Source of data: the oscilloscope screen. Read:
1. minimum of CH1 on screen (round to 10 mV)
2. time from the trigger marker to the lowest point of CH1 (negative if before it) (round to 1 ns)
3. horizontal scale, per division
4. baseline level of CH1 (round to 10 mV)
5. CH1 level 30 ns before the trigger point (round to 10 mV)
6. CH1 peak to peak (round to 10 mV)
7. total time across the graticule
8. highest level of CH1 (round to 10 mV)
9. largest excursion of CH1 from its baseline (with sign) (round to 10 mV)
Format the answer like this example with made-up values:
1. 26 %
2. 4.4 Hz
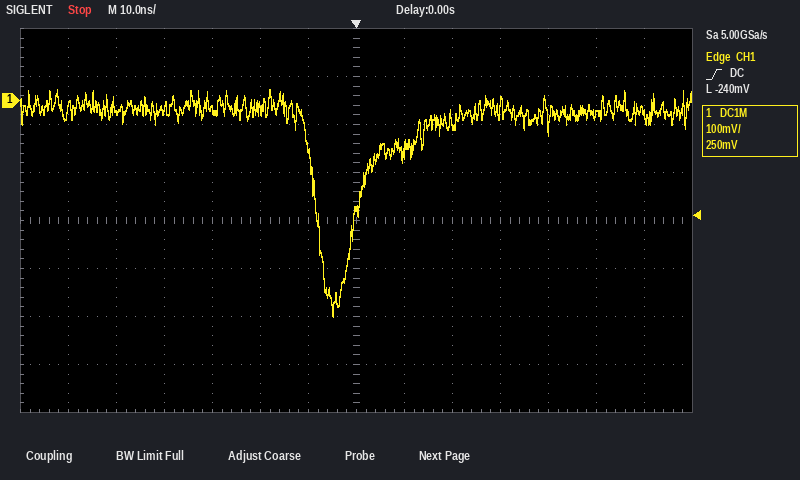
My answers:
1. -450 mV
2. -5 ns
3. 10 ns
4. -20 mV
5. -20 mV
6. 470 mV
7. 140 ns
8. 20 mV
9. -430 mV
